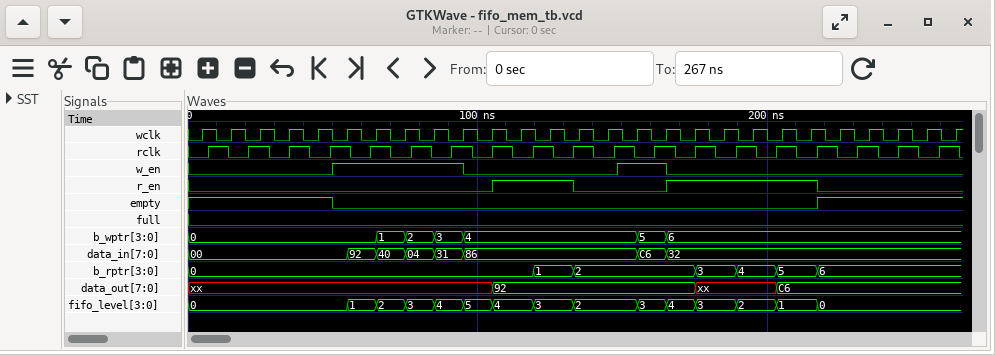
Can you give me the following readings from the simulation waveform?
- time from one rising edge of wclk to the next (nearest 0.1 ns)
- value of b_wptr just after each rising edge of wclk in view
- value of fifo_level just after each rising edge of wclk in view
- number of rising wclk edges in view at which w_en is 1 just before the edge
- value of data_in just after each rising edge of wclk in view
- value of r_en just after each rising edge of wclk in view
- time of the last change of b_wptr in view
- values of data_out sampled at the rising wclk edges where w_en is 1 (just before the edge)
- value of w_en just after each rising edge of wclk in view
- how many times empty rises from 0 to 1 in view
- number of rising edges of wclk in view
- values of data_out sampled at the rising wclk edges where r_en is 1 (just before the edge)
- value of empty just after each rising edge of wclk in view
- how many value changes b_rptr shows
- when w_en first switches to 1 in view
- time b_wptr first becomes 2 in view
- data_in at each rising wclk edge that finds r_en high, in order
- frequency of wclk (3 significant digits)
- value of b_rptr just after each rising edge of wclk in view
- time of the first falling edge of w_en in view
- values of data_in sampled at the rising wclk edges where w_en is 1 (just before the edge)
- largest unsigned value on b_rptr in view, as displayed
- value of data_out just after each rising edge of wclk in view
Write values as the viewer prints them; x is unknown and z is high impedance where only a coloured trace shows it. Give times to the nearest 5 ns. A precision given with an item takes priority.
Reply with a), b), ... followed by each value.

a) 10 ns
b) 0, 0, 0, 0, 0, 0, 1, 2, 3, 4, 4, 4, 4, 4, 4, 5, 6, 6, 6, 6, 6, 6, 6, 6, 6, 6, 6
c) 0, 0, 0, 0, 0, 1, 2, 3, 4, 5, 4, 4, 3, 2, 2, 3, 4, 3, 3, 2, 1, 1, 0, 0, 0, 0, 0
d) 7
e) 00, 00, 00, 00, 00, 92, 40, 04, 31, 86, 86, 86, 86, 86, 86, C6, 32, 32, 32, 32, 32, 32, 32, 32, 32, 32, 32
f) 0 0 0 0 0 0 0 0 0 0 1 1 1 0 0 0 1 1 1 1 1 1 0 0 0 0 0
g) 165 ns
h) xx, xx, xx, xx, xx, 92, 92
i) 0 0 0 0 0 1 1 1 1 0 0 0 0 0 0 1 0 0 0 0 0 0 0 0 0 0 0
j) 1
k) 27
l) 92, 92, 92, xx, xx, C6, C6
m) 1 1 1 1 1 0 0 0 0 0 0 0 0 0 0 0 0 0 0 0 0 0 1 1 1 1 1
n) 6
o) 50 ns
p) 75 ns
q) 86, 86, 32, 32, 32, 32, 32
r) 100 MHz
s) 0, 0, 0, 0, 0, 0, 0, 0, 0, 0, 0, 0, 1, 2, 2, 2, 2, 3, 3, 4, 5, 5, 6, 6, 6, 6, 6
t) 95 ns
u) 00, 92, 40, 04, 31, 86, C6
v) 6
w) xx, xx, xx, xx, xx, xx, xx, xx, xx, xx, 92, 92, 92, 92, 92, 92, 92, xx, xx, xx, C6, C6, C6, C6, C6, C6, C6
